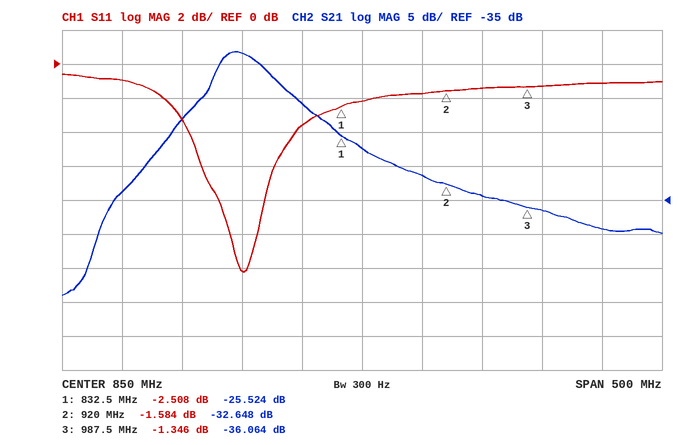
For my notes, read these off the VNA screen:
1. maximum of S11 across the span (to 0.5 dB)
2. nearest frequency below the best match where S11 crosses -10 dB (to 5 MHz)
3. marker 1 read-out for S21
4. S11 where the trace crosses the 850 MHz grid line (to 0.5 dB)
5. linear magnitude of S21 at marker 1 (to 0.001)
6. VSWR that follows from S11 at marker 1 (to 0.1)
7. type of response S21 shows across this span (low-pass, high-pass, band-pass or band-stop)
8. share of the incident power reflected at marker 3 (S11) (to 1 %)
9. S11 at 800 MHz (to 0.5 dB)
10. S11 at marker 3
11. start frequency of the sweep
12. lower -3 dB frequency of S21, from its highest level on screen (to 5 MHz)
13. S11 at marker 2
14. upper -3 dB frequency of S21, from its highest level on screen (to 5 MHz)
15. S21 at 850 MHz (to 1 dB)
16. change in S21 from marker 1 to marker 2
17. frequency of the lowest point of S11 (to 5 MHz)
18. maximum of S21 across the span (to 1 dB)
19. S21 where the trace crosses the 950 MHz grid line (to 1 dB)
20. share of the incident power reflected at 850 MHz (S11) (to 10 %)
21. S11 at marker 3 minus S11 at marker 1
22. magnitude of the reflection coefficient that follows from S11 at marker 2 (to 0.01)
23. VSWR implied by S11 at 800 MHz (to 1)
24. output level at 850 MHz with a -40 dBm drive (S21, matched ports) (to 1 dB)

-0.5 dB
740 MHz
-25.524 dB
-2.0 dB
0.053
7.0
band-pass
73 %
-3.5 dB
-1.346 dB
600 MHz
730 MHz
-1.584 dB
770 MHz
-27 dB
-7.124 dB
750 MHz
-13 dB
-34 dB
60 %
1.162 dB
0.83
5
-67 dBm
